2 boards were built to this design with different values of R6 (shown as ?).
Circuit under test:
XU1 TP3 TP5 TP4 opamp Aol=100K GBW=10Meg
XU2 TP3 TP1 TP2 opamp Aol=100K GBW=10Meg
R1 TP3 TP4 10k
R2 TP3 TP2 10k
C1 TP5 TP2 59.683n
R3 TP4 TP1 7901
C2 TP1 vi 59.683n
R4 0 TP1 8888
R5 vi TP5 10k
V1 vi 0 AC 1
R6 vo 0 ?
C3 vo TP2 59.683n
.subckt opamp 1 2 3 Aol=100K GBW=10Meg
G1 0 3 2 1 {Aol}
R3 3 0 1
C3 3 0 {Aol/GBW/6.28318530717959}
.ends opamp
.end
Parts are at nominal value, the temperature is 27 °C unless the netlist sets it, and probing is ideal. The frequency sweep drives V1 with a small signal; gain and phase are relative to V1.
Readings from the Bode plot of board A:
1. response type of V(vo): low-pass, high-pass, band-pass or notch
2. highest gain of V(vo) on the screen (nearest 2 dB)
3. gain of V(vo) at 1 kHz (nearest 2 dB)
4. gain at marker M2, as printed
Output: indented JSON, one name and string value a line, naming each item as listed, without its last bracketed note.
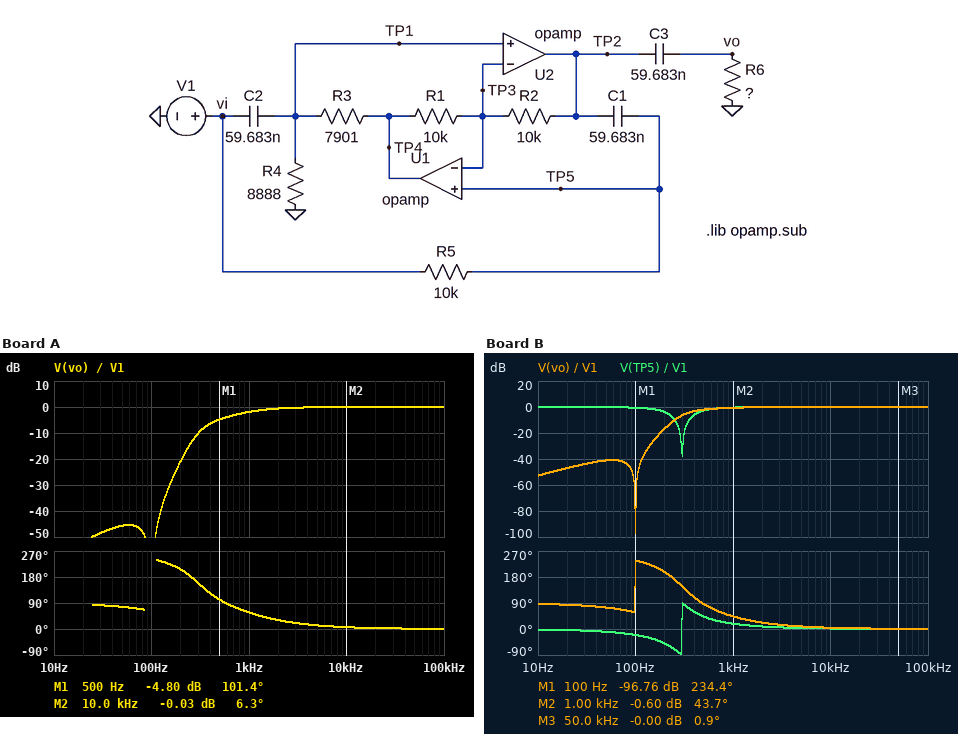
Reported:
{
  "response type of V(vo): low-pass, high-pass, band-pass or notch": "high-pass",
  "highest gain of V(vo) on the screen": "0 dB",
  "gain of V(vo) at 1 kHz": "-2 dB",
  "gain at marker M2, as printed": "-0.03 dB"
}
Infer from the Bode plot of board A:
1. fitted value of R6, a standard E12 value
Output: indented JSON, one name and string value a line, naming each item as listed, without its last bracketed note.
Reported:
{
  "fitted value of R6, a standard E12 value": "3.3 kΩ"
}
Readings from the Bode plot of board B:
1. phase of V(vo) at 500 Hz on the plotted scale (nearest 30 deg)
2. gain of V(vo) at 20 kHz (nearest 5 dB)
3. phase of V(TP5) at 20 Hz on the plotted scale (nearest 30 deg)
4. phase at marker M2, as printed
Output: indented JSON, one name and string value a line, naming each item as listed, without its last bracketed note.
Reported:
{
  "phase of V(vo) at 500 Hz on the plotted scale": "90 deg",
  "gain of V(vo) at 20 kHz": "0 dB",
  "phase of V(TP5) at 20 Hz on the plotted scale": "0 deg",
  "phase at marker M2, as printed": "43.7 deg"
}
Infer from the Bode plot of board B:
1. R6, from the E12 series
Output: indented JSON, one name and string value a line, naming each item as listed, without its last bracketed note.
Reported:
{
  "R6, from the E12 series": "5.6 kΩ"
}
